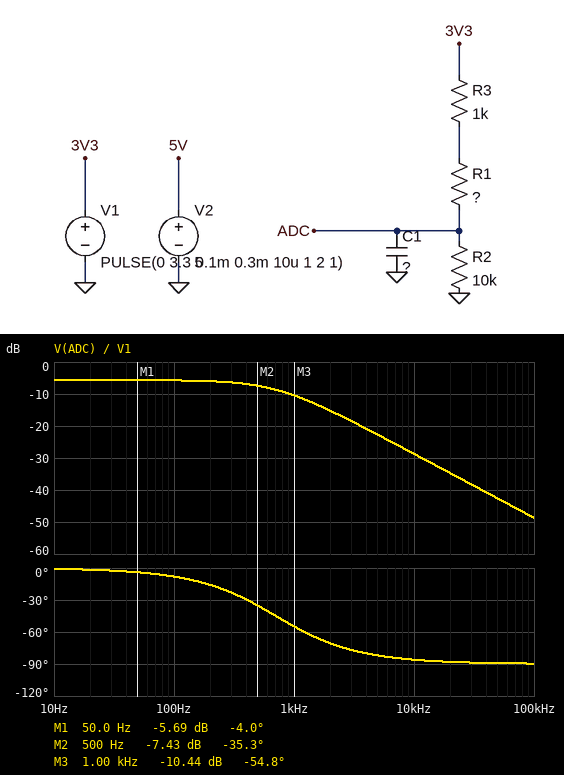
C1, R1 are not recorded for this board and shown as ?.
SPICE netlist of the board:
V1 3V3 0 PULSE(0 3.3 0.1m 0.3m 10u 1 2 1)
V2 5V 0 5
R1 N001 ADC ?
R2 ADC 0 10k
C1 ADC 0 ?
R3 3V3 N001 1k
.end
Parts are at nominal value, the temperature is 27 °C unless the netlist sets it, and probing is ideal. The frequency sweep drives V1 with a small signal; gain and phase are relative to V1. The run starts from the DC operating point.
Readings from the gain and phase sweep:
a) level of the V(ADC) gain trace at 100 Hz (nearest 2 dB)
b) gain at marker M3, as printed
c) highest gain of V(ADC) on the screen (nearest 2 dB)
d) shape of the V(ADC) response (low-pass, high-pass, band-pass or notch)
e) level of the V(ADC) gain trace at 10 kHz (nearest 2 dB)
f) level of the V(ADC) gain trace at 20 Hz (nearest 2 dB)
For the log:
-6 dB
-10.44 dB
-6 dB
low-pass
-28 dB
-6 dB
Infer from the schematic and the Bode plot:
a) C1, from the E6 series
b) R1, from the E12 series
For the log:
47 nF
8.2 kΩ
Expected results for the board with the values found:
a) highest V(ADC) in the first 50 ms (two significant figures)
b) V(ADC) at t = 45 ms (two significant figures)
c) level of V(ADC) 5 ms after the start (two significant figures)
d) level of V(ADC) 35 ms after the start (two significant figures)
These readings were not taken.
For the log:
1.7 V
1.7 V
1.7 V
1.7 V
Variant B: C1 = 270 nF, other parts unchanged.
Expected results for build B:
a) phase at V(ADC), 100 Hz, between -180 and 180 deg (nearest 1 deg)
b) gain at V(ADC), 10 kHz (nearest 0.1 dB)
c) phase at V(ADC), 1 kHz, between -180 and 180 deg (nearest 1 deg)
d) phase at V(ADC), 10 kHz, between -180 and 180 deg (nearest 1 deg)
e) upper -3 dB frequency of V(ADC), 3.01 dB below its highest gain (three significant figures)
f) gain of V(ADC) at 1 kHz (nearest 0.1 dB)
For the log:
-39 deg
-43.9 dB
-83 deg
-89 deg
123 Hz
-23.9 dB
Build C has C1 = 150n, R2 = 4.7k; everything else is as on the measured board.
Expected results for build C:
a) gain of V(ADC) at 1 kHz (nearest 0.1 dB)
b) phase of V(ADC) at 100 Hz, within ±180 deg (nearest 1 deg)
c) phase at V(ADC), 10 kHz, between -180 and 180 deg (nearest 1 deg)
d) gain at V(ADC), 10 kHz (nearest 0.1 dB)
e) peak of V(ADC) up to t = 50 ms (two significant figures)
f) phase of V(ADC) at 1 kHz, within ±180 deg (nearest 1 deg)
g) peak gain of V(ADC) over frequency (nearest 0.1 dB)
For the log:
-19.2 dB
-16 deg
-88 deg
-38.8 dB
1.1 V
-71 deg
-9.4 dB
